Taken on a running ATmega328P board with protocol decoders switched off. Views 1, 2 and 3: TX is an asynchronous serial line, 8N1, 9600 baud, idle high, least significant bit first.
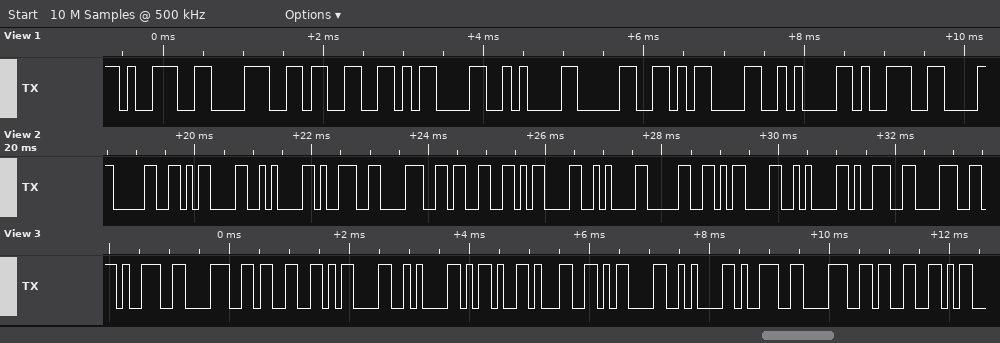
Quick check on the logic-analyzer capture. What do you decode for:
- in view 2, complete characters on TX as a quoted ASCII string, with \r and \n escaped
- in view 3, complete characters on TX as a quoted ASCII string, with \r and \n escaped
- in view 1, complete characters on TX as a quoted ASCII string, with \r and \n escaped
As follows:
"0\r\n983\r\n0\r\n98"
"983\r\n-1\r\n983"
"983\r\n0\r\n9"
